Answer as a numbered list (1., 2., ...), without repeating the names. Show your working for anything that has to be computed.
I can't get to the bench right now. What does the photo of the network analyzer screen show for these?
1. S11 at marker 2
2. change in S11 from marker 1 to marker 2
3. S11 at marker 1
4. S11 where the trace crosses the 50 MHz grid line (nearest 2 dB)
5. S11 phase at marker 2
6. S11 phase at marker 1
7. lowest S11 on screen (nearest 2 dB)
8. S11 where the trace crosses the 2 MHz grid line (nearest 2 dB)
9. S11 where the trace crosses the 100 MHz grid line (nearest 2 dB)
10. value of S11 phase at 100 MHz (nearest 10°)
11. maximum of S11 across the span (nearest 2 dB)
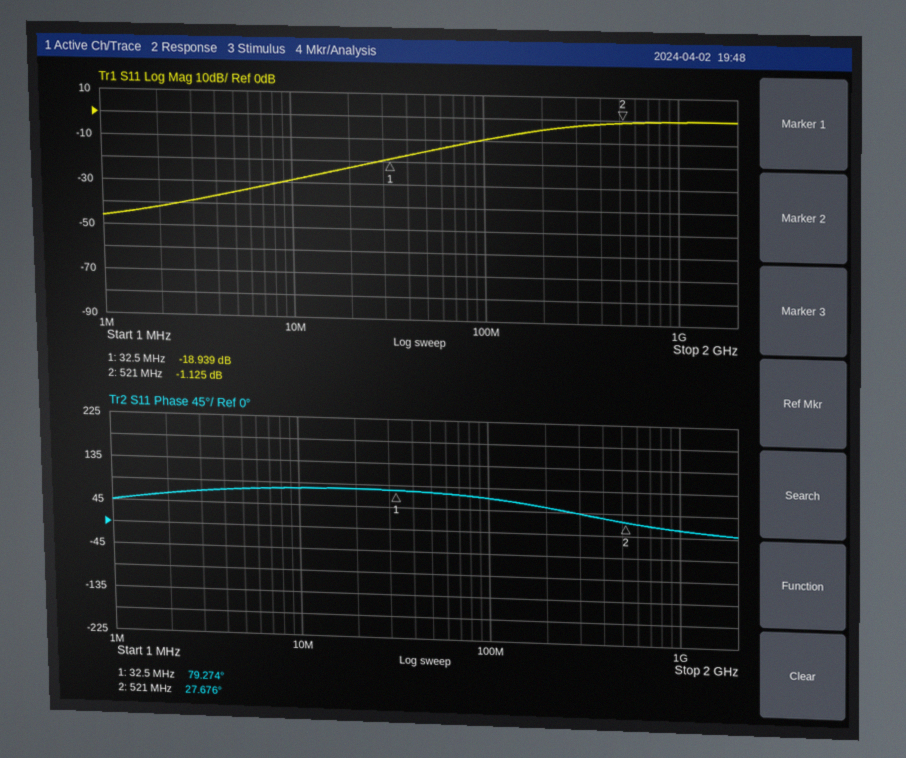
1. -1.125 dB
2. -1.125 − (-18.939) = 17.814 dB
3. -18.939 dB
4. -16 dB
5. 27.676°
6. 79.274°
7. -46 dB
8. -42 dB
9. -10 dB
10. 70°
11. 0 dB
